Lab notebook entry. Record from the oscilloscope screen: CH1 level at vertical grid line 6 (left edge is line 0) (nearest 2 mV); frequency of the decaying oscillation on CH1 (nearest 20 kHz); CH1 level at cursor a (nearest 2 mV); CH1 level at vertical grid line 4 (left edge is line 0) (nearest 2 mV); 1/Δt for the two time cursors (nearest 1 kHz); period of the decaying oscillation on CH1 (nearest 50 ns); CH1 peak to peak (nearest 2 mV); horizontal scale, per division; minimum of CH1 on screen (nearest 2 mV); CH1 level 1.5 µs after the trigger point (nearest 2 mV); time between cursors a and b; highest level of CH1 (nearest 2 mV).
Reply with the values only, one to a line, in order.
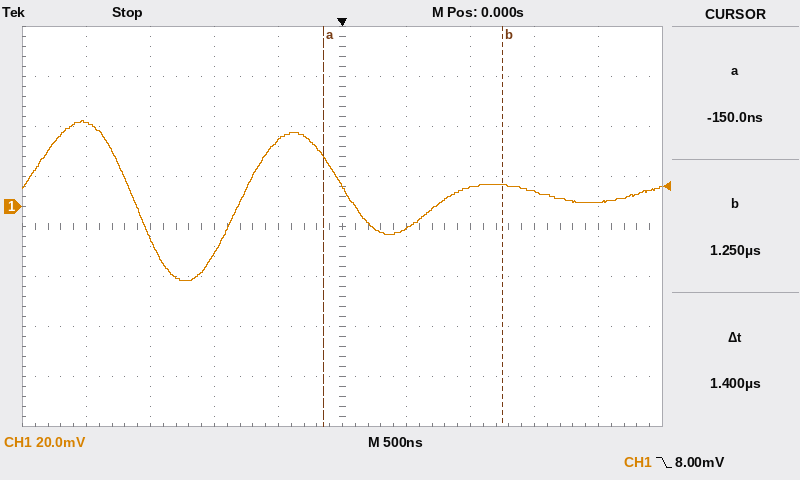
-8 mV
620 kHz
20 mV
26 mV
714 kHz
1.60 µs
64 mV
500 ns
-30 mV
6 mV
1.4 µs
34 mV
